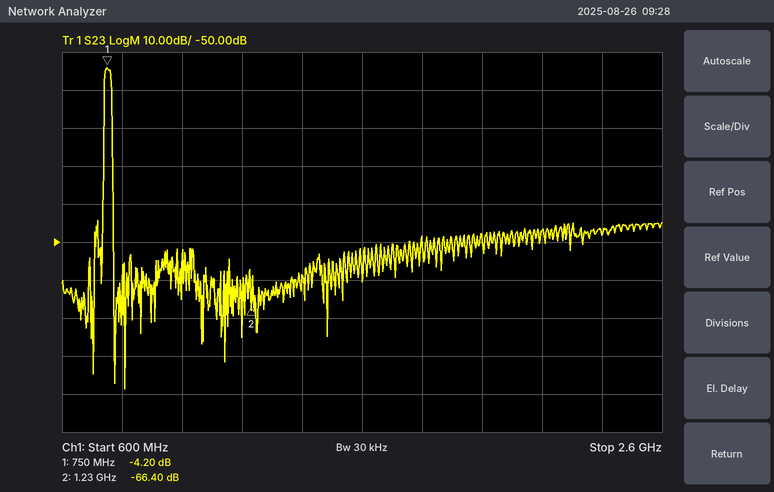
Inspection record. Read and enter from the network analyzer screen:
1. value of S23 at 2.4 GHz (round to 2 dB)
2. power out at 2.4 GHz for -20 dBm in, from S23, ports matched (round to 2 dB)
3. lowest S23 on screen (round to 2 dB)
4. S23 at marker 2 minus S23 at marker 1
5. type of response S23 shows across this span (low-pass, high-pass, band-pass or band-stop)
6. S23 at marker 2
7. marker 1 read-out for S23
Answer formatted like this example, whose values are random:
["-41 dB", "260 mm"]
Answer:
["-48 dB", "-68 dBm", "-88 dB", "-62.20 dB", "band-pass", "-66.40 dB", "-4.20 dB"]
